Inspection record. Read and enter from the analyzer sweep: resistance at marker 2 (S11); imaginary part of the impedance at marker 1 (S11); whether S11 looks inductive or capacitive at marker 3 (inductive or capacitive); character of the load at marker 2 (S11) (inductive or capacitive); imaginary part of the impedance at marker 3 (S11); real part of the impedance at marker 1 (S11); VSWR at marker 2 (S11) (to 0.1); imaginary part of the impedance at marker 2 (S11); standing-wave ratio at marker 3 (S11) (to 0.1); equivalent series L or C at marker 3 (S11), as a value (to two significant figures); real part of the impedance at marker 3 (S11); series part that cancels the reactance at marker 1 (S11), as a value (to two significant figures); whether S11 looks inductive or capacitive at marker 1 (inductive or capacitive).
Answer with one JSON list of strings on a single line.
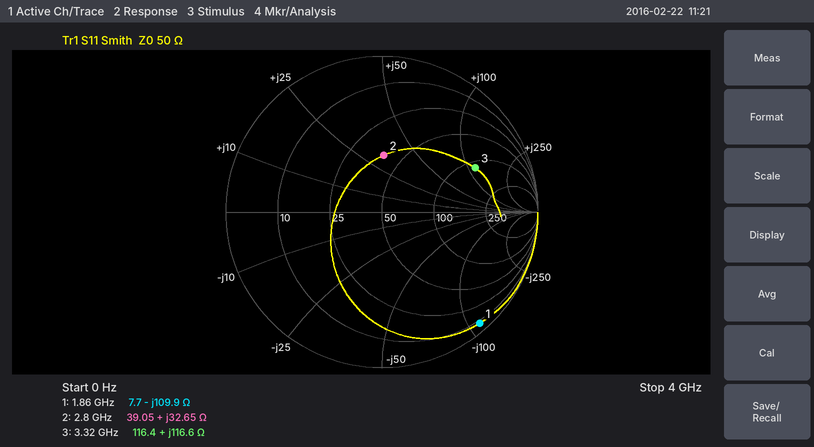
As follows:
["39.05 Ω", "-109.9 Ω", "inductive", "inductive", "+116.6 Ω", "7.7 Ω", "2.1", "+32.65 Ω", "4.9", "5.6 nH", "116.4 Ω", "9.4 nH", "capacitive"]
